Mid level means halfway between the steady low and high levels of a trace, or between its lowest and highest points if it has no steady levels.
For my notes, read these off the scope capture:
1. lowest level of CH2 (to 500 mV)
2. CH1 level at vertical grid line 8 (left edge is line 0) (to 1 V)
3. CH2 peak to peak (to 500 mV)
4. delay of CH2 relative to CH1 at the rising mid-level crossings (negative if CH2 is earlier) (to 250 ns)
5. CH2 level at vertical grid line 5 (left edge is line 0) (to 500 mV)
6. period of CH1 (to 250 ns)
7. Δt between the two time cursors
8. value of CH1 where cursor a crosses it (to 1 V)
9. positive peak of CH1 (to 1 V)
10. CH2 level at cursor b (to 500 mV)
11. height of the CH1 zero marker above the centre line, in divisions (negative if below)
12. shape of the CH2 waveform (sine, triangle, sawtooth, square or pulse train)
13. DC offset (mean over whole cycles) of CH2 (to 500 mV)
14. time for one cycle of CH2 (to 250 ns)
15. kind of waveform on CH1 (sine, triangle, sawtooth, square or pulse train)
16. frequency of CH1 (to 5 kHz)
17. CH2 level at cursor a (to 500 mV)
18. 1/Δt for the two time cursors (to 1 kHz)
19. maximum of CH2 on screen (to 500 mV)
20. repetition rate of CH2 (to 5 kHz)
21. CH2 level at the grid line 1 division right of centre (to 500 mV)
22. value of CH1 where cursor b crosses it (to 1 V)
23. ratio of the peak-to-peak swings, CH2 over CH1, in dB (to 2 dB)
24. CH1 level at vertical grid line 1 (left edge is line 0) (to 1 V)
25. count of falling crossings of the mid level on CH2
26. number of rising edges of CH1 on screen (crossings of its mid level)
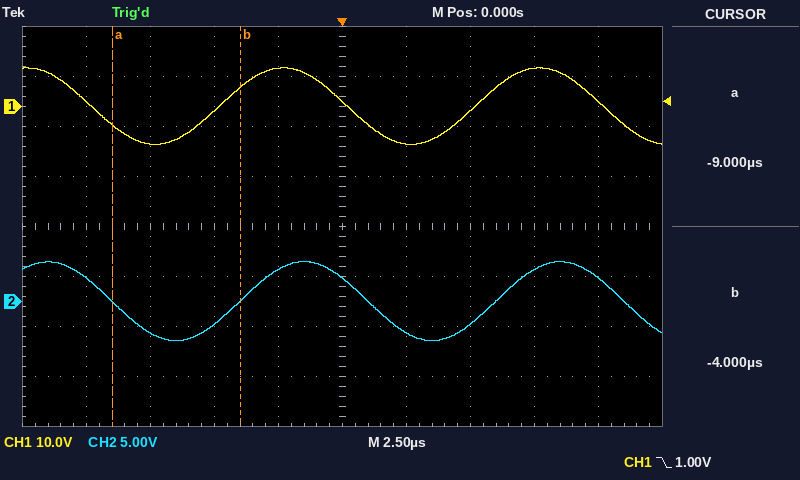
-4.0 V
8 V
8.0 V
+750 ns
2.5 V
10.00 µs
5.00 µs
-4 V
8 V
0.0 V
+2.4 div
sine
0.0 V
10.00 µs
sine
100 kHz
0.0 V
200 kHz
4.0 V
100 kHz
-3.0 V
4 V
-6 dB
1 V
3
2
